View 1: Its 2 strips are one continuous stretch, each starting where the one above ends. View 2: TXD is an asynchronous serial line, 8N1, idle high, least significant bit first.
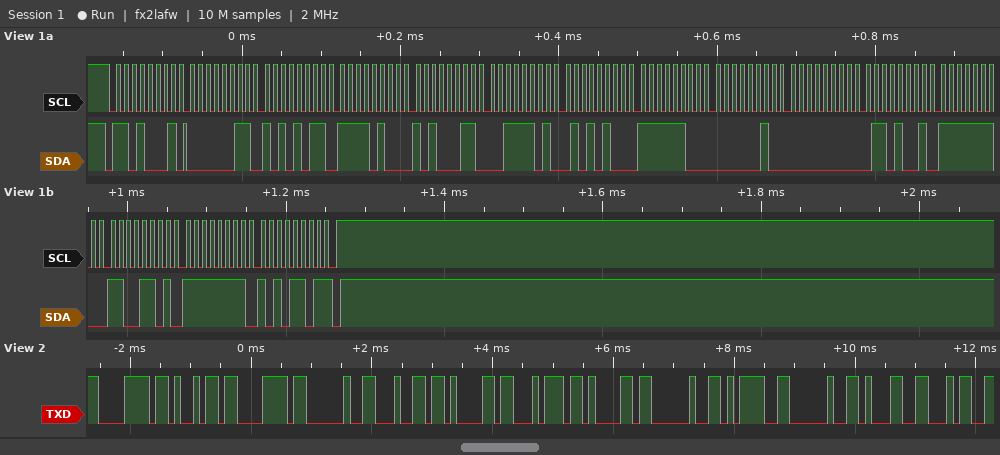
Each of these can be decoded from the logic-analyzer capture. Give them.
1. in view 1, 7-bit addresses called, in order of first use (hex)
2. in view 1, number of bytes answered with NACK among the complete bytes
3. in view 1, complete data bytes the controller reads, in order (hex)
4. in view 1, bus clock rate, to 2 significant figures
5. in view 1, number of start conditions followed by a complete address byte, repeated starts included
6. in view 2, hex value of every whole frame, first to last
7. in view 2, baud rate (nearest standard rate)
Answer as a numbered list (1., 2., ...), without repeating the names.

1. 0x68
2. 1
3. 03 AB F4 A3 3D 54 FC 02 00 69 FE CD FF AD
4. 100 kHz
5. 1
6. 78 69 78 20 64 61 74 61 20 3D 20 31 34
7. 9600 baud
